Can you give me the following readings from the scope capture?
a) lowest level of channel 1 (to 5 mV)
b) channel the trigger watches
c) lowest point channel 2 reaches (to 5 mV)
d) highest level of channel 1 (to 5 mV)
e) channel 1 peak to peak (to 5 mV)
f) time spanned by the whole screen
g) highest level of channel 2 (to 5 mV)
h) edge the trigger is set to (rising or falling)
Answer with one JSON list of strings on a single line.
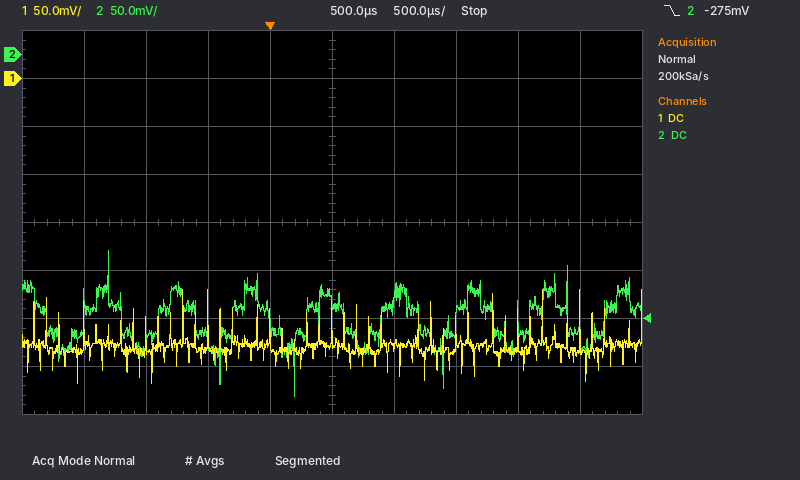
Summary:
["-320 mV", "channel 2", "-355 mV", "-220 mV", "100 mV", "5 ms", "-205 mV", "falling"]
